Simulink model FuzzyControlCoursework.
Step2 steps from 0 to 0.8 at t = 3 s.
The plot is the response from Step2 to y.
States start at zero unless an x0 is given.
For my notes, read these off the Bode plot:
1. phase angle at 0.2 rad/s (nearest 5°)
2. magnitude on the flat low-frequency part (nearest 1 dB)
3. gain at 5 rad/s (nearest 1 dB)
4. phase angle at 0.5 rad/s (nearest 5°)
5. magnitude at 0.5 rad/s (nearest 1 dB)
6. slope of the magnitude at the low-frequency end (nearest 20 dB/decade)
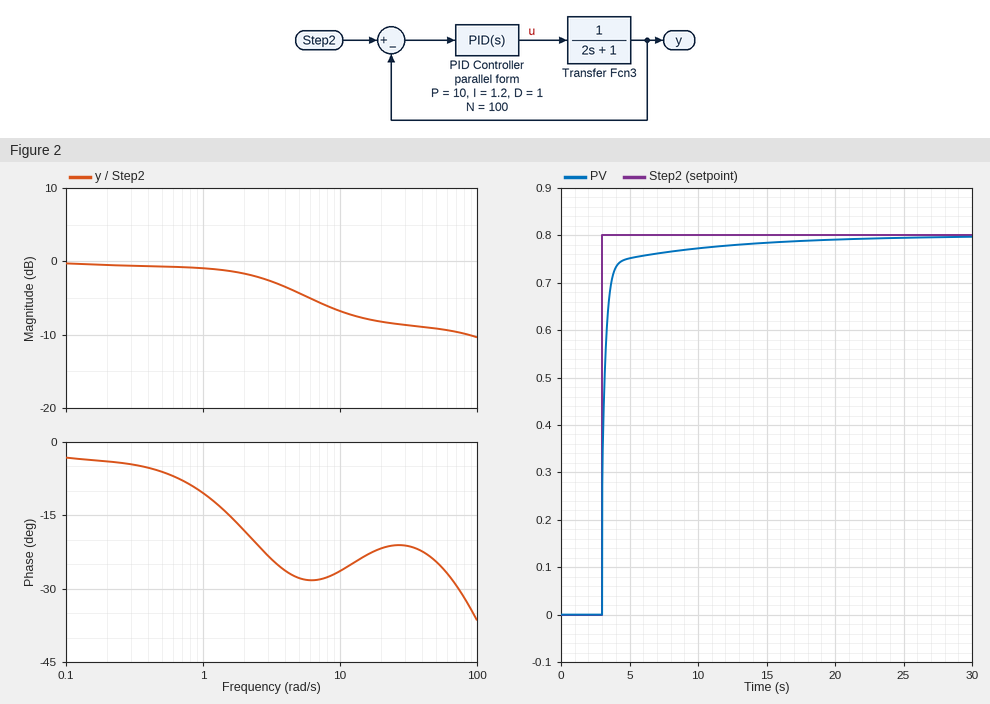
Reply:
-5°
0 dB
-4 dB
-5°
-1 dB
0 dB/decade
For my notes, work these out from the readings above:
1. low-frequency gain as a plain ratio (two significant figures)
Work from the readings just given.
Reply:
1.0
